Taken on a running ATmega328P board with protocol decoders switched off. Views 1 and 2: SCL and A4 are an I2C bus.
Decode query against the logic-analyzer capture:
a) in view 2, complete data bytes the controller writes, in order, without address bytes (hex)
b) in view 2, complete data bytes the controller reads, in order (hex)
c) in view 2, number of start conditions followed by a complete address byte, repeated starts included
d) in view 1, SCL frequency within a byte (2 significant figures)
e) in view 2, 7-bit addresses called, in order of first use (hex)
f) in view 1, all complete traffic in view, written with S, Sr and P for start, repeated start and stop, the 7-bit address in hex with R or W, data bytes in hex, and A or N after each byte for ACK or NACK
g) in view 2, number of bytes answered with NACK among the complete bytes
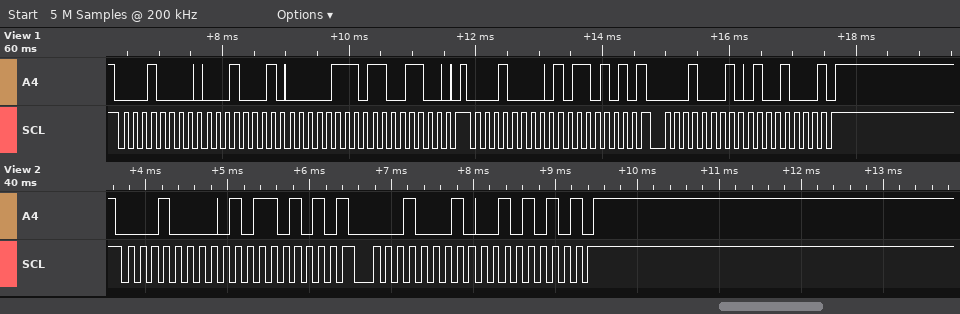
B5
2A
2
6.9 kHz
0x08
S 08W A 11 A 07 A CC A P S 08W A B5 A Sr 08R A 48 N P
1
